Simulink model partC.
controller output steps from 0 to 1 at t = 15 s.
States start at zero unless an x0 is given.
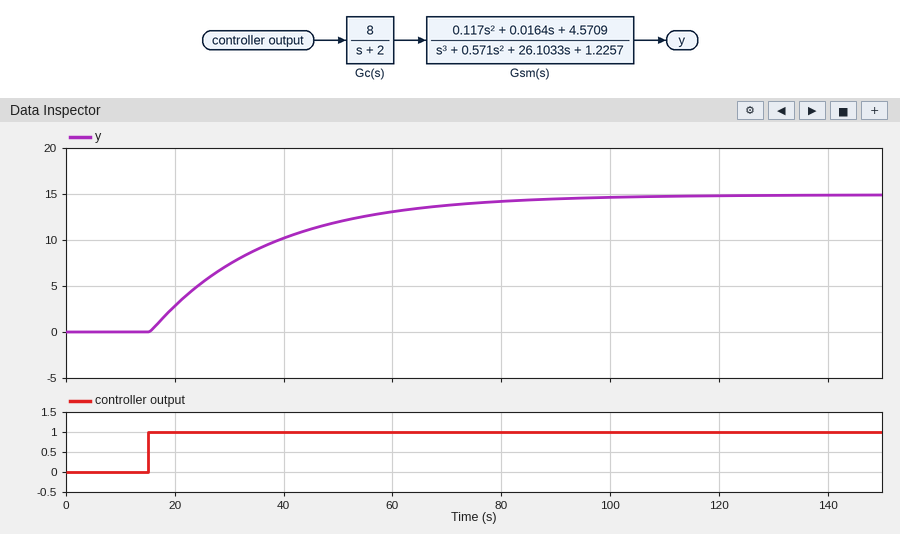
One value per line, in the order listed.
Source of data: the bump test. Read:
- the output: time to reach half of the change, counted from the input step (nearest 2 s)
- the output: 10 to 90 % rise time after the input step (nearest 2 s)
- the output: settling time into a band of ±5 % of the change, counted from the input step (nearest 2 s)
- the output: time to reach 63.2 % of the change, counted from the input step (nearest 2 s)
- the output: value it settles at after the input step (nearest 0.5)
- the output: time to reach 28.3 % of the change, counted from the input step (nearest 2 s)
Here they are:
16 s
46 s
64 s
22 s
15.0
8 s
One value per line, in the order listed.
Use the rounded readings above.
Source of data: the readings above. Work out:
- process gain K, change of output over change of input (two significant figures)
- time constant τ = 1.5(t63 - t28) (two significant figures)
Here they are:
15
21 s
